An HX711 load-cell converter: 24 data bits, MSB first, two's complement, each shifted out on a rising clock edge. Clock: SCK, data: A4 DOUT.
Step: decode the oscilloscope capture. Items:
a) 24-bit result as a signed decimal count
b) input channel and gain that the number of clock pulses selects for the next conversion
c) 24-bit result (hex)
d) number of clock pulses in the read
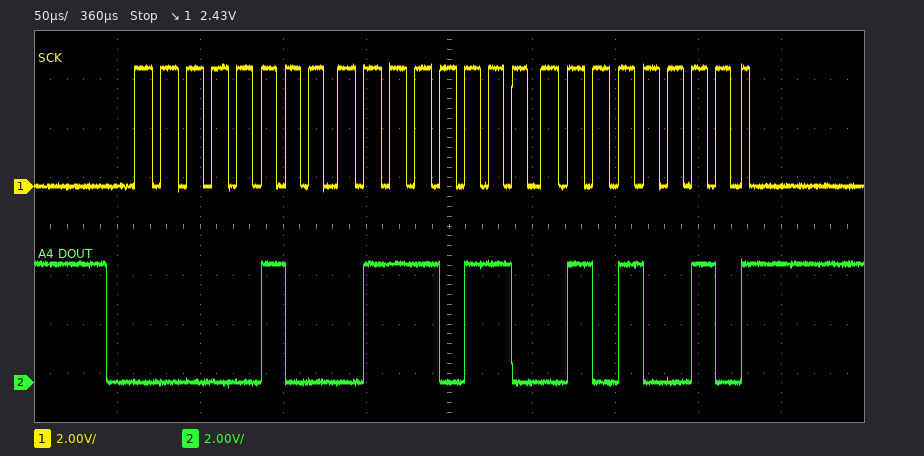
292434
channel A, gain 128
0x047652
25
